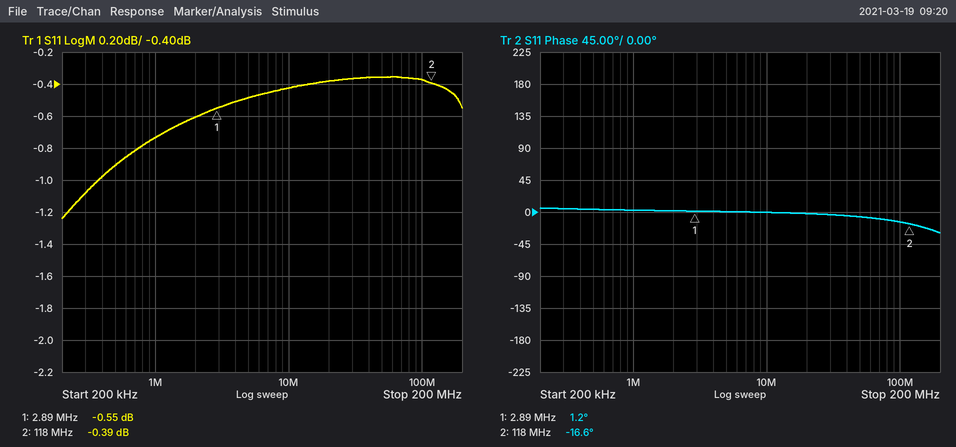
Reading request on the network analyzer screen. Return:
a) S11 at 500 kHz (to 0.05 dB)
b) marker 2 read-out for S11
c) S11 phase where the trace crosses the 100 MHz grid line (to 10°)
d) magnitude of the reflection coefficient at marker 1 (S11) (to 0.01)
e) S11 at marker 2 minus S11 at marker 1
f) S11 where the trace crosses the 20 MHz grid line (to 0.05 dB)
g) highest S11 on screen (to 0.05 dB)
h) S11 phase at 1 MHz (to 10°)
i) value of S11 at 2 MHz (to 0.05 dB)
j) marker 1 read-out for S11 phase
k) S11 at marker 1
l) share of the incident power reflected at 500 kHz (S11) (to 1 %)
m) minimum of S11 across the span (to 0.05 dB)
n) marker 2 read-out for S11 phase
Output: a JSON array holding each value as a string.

["-0.90 dB", "-0.39 dB", "-10°", "0.94", "0.16 dB", "-0.40 dB", "-0.35 dB", "0°", "-0.60 dB", "1.2°", "-0.55 dB", "81 %", "-1.25 dB", "-16.6°"]
